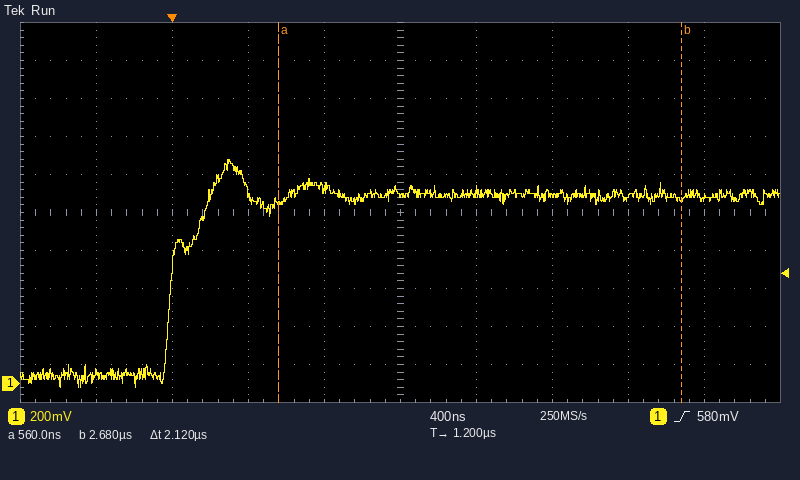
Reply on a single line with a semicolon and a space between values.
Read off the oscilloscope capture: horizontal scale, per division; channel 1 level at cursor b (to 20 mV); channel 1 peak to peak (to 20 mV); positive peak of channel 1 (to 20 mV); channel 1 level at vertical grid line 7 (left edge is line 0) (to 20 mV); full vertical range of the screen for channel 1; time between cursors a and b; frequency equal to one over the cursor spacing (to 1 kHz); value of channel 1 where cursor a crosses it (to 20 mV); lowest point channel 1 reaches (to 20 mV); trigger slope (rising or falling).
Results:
400 ns; 980 mV; 1.20 V; 1.18 V; 1.00 V; 2 V; 2.12 µs; 472 kHz; 960 mV; -20 mV; rising
